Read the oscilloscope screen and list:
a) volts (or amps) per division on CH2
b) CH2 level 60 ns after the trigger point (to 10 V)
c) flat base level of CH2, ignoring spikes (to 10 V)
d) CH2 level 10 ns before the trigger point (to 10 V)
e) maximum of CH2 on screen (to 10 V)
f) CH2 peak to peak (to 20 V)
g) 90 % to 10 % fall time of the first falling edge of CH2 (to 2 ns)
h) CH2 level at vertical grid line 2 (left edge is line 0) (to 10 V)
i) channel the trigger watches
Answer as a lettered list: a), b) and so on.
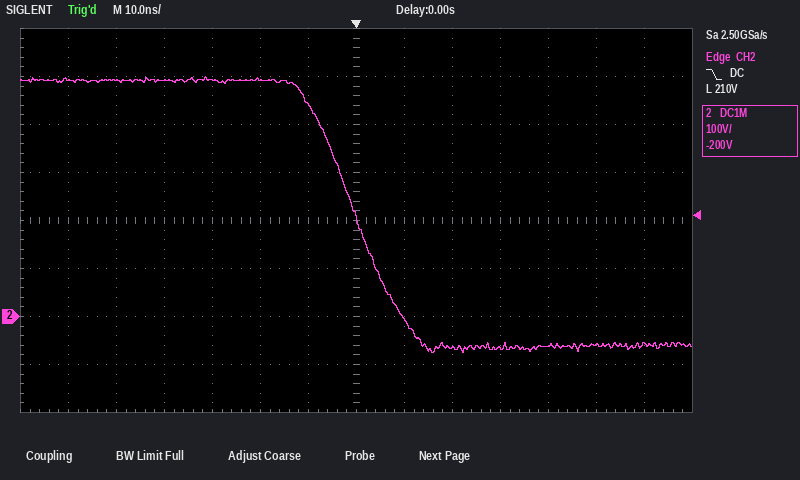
a) 100 V
b) -60 V
c) -60 V
d) 440 V
e) 500 V
f) 580 V
g) 20 ns
h) 490 V
i) CH2
